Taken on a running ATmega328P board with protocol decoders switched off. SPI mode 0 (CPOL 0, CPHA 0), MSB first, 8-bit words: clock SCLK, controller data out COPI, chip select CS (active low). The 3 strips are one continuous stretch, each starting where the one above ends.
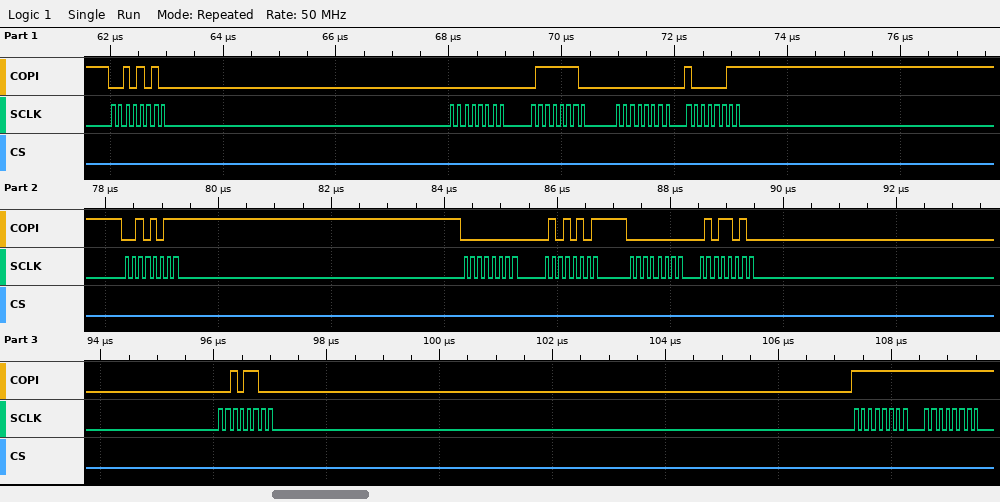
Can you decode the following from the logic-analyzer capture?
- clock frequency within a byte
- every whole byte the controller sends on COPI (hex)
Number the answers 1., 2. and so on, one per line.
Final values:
1. 8 MHz
2. 2A 00 7E 00 83 2B 00 55 00 5A 2C FF FF
